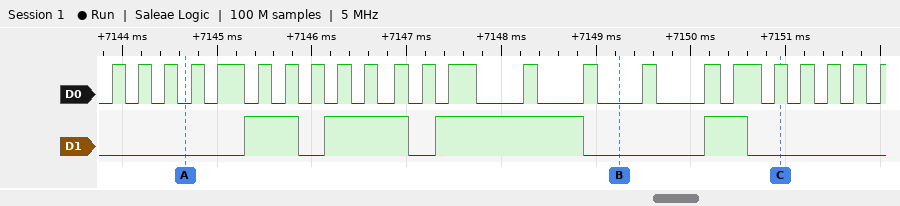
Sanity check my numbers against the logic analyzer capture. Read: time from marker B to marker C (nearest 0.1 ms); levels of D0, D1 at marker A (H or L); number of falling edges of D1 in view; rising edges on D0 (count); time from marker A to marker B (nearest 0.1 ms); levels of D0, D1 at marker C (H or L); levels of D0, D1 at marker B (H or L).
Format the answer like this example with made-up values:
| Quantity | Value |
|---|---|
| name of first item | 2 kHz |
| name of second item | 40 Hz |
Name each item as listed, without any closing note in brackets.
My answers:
| Quantity | Value |
|---|---|
| time from marker B to marker C | 1.7 ms |
| levels of D0, D1 at marker A | D0=L, D1=L |
| number of falling edges of D1 in view | 4 |
| rising edges on D0 | 23 |
| time from marker A to marker B | 4.6 ms |
| levels of D0, D1 at marker C | D0=H, D1=L |
| levels of D0, D1 at marker B | D0=L, D1=L |
